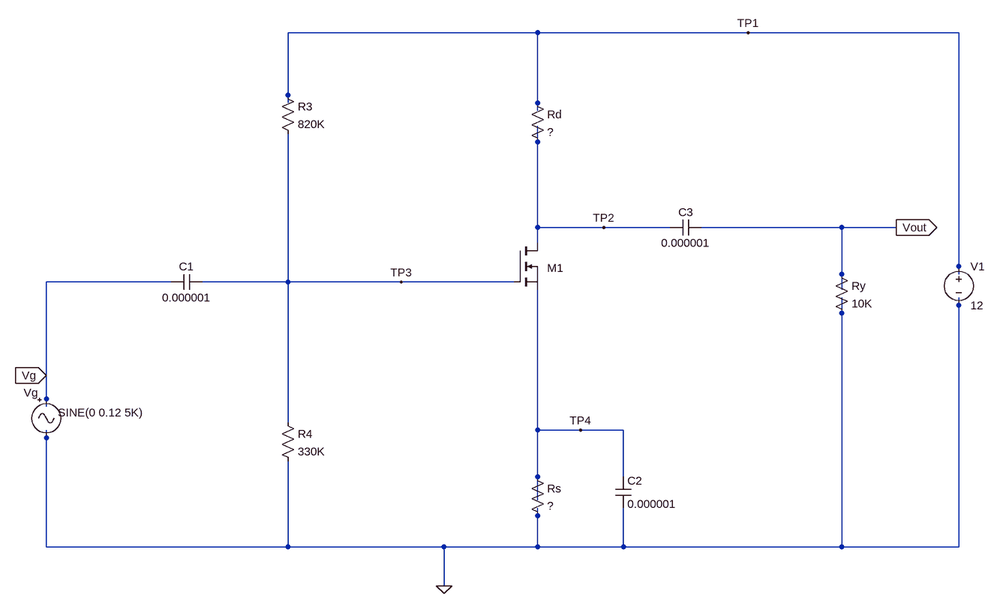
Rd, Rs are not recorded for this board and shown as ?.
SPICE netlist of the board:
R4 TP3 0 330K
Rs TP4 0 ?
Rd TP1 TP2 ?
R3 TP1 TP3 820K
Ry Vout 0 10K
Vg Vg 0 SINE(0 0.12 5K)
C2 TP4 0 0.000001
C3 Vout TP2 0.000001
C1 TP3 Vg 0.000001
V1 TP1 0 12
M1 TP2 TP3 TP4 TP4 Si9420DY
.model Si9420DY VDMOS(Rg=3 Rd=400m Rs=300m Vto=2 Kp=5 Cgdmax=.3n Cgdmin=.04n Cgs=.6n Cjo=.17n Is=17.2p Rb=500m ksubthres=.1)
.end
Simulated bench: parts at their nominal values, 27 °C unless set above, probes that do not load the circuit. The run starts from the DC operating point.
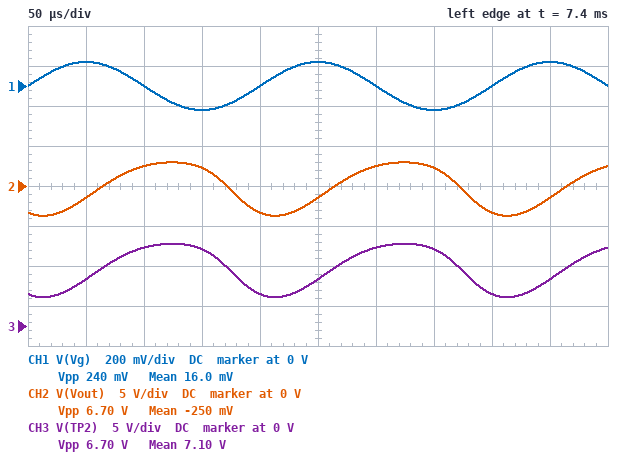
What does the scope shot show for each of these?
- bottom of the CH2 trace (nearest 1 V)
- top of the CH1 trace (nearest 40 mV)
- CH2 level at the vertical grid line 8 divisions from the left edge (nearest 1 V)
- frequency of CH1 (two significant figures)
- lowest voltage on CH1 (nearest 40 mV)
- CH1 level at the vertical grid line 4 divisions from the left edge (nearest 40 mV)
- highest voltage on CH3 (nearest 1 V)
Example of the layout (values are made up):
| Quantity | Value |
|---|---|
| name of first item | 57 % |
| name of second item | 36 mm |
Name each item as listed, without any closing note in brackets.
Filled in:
| Quantity | Value |
|---|---|
| bottom of the CH2 trace | -4 V |
| top of the CH1 trace | 120 mV |
| CH2 level at the vertical grid line 8 divisions from the left edge | -3 V |
| frequency of CH1 | 5.0 kHz |
| lowest voltage on CH1 | -120 mV |
| CH1 level at the vertical grid line 4 divisions from the left edge | 0 V |
| highest voltage on CH3 | 10 V |
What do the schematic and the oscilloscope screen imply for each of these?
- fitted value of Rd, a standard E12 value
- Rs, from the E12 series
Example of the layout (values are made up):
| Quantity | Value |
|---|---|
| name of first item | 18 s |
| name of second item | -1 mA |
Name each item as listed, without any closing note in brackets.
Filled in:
| Quantity | Value |
|---|---|
| fitted value of Rd, a standard E12 value | 1.2 kΩ |
| Rs, from the E12 series | 390 Ω |
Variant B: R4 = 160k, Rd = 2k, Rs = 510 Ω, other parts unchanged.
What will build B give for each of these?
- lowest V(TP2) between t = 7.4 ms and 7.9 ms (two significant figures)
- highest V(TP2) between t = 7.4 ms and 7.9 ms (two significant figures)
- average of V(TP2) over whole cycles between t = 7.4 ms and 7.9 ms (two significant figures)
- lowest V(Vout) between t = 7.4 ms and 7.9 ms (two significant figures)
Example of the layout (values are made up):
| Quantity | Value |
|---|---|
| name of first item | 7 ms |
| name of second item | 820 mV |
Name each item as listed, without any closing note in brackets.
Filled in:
| Quantity | Value |
|---|---|
| lowest V(TP2) between t = 7.4 ms and 7.9 ms | 9.6 V |
| highest V(TP2) between t = 7.4 ms and 7.9 ms | 12 V |
| average of V(TP2) over whole cycles between t = 7.4 ms and 7.9 ms | 11 V |
| lowest V(Vout) between t = 7.4 ms and 7.9 ms | -1.7 V |
